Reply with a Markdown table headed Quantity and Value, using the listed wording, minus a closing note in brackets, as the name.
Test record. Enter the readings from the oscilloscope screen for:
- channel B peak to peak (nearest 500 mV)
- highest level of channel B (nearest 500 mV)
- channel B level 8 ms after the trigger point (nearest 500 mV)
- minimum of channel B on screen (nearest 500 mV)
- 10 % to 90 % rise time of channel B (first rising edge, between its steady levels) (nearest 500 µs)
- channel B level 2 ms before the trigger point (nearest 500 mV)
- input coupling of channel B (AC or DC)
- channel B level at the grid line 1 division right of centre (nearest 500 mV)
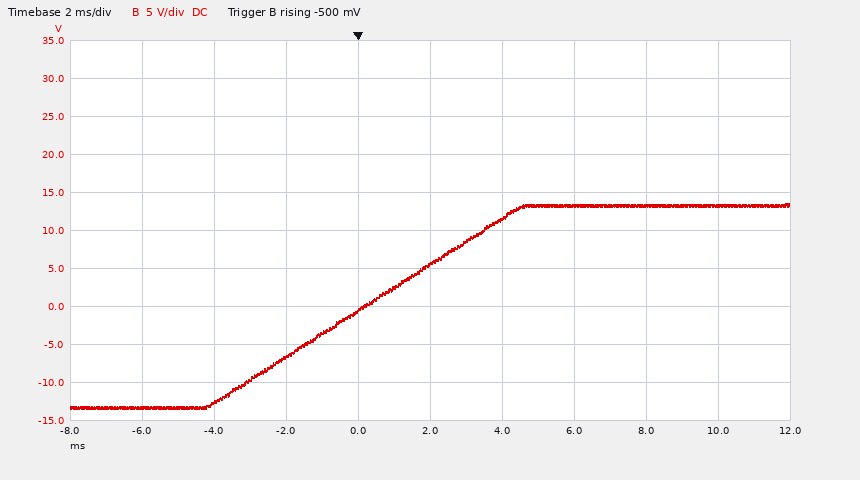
| Quantity | Value |
|---|---|
| channel B peak to peak | 27.0 V |
| highest level of channel B | 13.5 V |
| channel B level 8 ms after the trigger point | 13.5 V |
| minimum of channel B on screen | -13.5 V |
| 10 % to 90 % rise time of channel B (first rising edge, between its steady levels) | 7.0 ms |
| channel B level 2 ms before the trigger point | -6.5 V |
| input coupling of channel B | DC |
| channel B level at the grid line 1 division right of centre | 11.5 V |
